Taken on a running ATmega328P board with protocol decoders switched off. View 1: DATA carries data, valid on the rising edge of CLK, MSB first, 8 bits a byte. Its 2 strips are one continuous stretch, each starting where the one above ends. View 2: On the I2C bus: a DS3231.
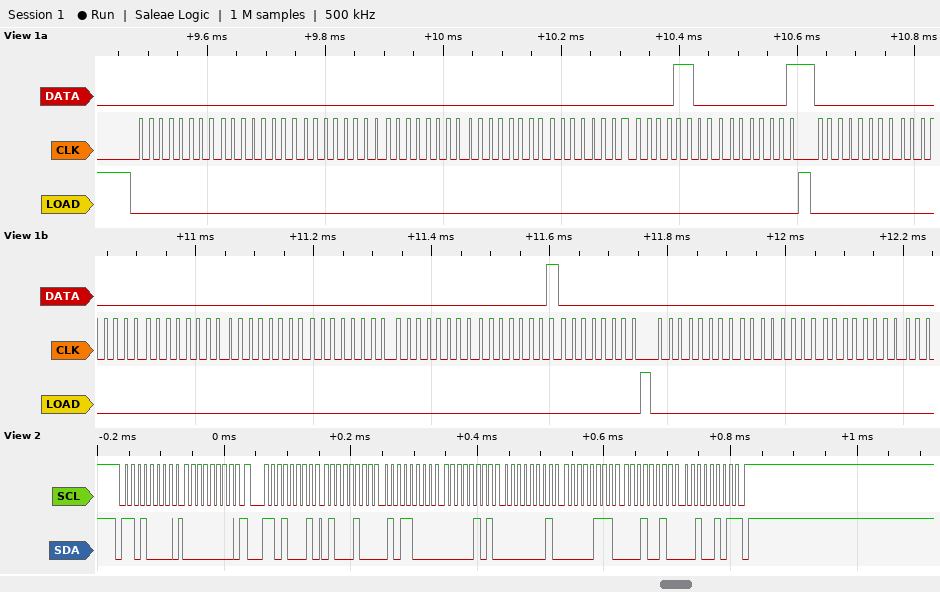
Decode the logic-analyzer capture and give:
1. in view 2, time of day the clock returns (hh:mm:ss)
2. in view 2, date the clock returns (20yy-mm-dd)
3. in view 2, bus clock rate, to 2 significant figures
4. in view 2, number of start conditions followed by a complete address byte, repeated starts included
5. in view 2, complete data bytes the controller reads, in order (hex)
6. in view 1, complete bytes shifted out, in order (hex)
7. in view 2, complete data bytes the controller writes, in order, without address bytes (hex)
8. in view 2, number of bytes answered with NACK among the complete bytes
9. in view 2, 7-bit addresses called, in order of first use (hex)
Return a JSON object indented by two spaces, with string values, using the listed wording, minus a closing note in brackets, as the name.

{
  "in view 2, time of day the clock returns": "05:58:44",
  "in view 2, date the clock returns": "2025-12-07",
  "in view 2, bus clock rate, to 2 significant figures": "100 kHz",
  "in view 2, number of start conditions followed by a complete address byte, repeated starts included": "2",
  "in view 2, complete data bytes the controller reads, in order": "44 58 05 01 07 12 25",
  "in view 1, complete bytes shifted out, in order": "0x00 0x00 0x00 0x00 0x00 0x00 0x0C 0x01 0x00 0x00 0x00 0x00 0x00 0x00 0x01 0x00 0x00 0x00 0x00",
  "in view 2, complete data bytes the controller writes, in order, without address bytes": "00",
  "in view 2, number of bytes answered with NACK among the complete bytes": "1",
  "in view 2, 7-bit addresses called, in order of first use": "0x68"
}
